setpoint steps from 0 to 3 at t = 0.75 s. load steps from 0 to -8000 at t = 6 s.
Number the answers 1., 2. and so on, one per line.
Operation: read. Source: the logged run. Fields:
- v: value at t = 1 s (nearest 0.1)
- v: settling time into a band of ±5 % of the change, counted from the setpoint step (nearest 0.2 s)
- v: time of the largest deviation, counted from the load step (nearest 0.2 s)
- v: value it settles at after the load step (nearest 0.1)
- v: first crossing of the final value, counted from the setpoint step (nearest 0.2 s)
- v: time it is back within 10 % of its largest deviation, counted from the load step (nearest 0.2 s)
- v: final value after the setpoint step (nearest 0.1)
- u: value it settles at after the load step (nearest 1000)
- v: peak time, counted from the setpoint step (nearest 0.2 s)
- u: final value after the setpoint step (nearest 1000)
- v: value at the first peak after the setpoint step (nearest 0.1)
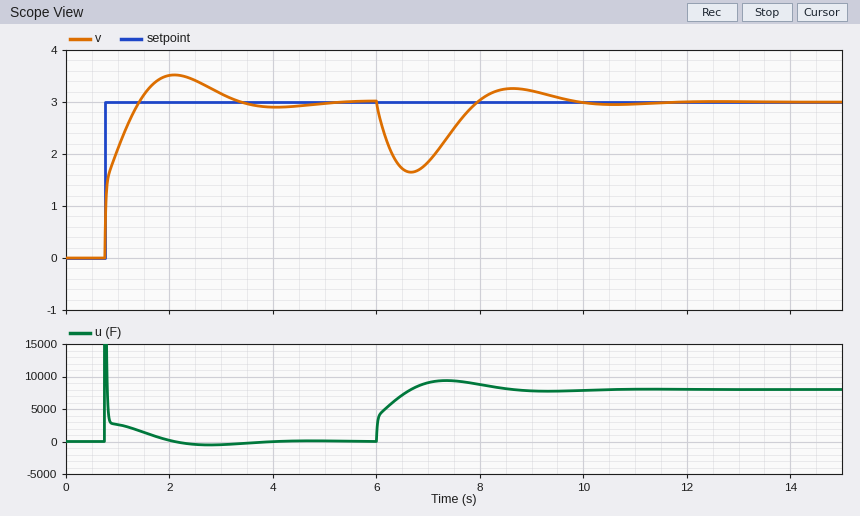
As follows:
1. 2.1
2. 2.2 s
3. 0.6 s
4. 3.0
5. 0.6 s
6. 3.4 s
7. 3.0
8. 8000
9. 1.4 s
10. 0
11. 3.5
